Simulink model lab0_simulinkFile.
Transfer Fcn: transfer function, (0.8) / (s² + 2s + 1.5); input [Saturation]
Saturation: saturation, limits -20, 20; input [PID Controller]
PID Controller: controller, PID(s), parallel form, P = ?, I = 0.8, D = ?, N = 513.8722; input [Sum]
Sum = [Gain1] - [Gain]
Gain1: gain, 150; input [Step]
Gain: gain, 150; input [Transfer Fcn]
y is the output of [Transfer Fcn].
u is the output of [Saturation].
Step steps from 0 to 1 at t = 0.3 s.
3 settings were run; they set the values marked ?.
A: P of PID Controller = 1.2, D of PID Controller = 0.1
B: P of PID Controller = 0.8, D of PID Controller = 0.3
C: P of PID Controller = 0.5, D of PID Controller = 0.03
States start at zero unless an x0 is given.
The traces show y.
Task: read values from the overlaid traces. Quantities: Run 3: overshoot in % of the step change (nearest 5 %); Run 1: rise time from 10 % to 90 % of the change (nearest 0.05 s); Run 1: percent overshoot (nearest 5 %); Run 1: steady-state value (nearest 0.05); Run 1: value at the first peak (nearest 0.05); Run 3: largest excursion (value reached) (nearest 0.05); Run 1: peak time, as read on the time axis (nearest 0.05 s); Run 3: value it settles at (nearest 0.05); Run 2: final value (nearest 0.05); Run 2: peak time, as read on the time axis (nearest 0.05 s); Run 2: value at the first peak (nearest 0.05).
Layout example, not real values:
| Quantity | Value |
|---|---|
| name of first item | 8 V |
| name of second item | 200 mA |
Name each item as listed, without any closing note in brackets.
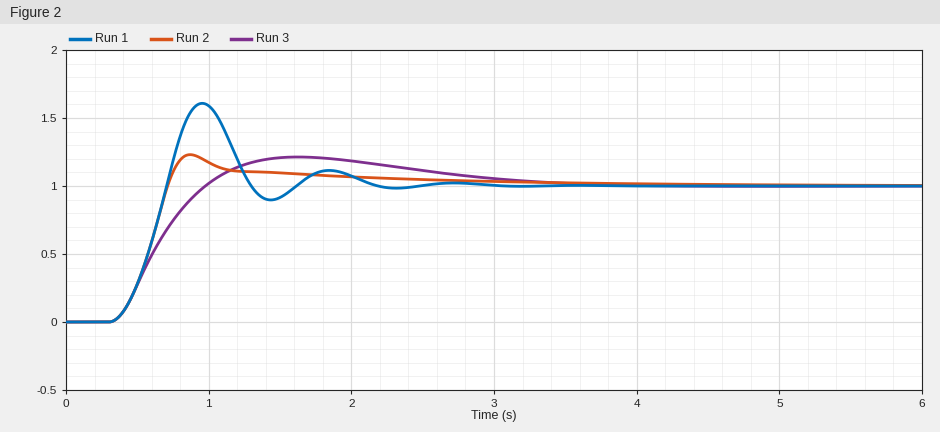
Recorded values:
| Quantity | Value |
|---|---|
| Run 3: overshoot in % of the step change | 20 % |
| Run 1: rise time from 10 % to 90 % of the change | 0.25 s |
| Run 1: percent overshoot | 60 % |
| Run 1: steady-state value | 1.00 |
| Run 1: value at the first peak | 1.60 |
| Run 3: largest excursion (value reached) | 1.20 |
| Run 1: peak time, as read on the time axis | 0.95 s |
| Run 3: value it settles at | 1.00 |
| Run 2: final value | 1.00 |
| Run 2: peak time, as read on the time axis | 0.85 s |
| Run 2: value at the first peak | 1.25 |
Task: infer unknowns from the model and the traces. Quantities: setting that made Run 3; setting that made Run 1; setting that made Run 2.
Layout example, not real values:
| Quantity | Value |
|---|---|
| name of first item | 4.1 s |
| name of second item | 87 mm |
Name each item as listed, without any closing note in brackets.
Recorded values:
| Quantity | Value |
|---|---|
| setting that made Run 3 | B |
| setting that made Run 1 | C |
| setting that made Run 2 | A |
